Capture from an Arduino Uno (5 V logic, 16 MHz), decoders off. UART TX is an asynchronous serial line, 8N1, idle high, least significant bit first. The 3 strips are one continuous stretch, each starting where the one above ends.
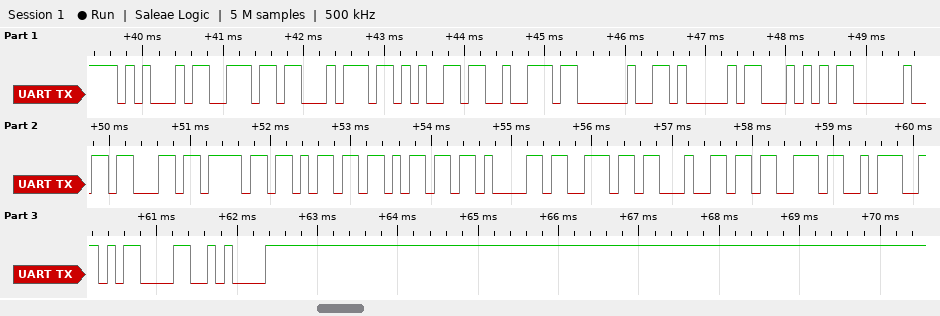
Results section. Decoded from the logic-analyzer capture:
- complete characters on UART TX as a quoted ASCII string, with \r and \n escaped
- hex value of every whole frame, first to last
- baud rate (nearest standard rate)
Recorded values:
"Enter AT commands:\r\n"
0x45 0x6E 0x74 0x65 0x72 0x20 0x41 0x54 0x20 0x63 0x6F 0x6D 0x6D 0x61 0x6E 0x64 0x73 0x3A 0x0D 0x0A
9600 baud
